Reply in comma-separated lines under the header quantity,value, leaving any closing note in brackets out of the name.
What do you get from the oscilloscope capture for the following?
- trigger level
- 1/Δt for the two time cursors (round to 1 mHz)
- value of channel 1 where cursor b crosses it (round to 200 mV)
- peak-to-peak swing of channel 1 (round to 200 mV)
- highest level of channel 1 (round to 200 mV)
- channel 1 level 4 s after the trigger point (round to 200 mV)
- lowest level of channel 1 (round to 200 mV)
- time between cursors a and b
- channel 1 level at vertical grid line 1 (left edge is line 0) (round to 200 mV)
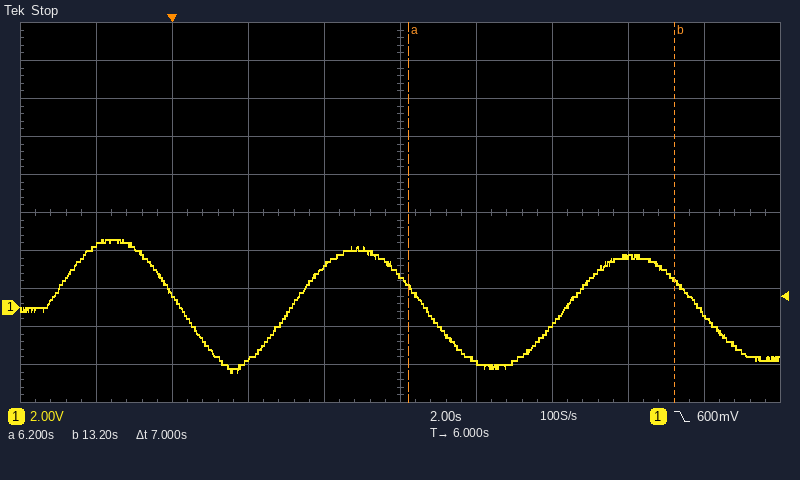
quantity,value
trigger level,600 mV
1/Δt for the two time cursors,143 mHz
value of channel 1 where cursor b crosses it,1.4 V
peak-to-peak swing of channel 1,7.0 V
highest level of channel 1,3.6 V
channel 1 level 4 s after the trigger point,2.2 V
lowest level of channel 1,-3.4 V
time between cursors a and b,7 s
channel 1 level at vertical grid line 1 (left edge is line 0),3.2 V
